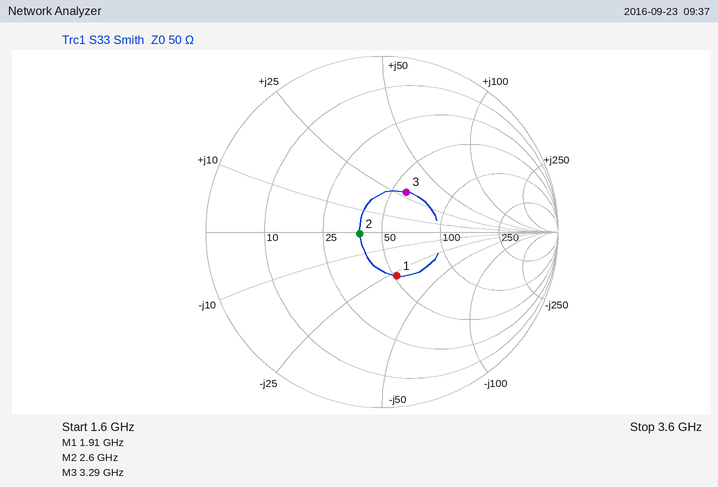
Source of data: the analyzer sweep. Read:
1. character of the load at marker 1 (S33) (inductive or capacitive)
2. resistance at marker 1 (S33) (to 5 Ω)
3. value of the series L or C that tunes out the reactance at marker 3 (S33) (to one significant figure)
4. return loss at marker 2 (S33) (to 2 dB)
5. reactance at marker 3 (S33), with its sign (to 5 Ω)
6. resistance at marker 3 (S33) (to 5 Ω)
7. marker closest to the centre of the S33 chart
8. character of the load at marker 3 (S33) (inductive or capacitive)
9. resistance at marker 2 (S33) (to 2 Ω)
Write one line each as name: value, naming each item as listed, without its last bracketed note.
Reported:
character of the load at marker 1 (S33): capacitive
resistance at marker 1 (S33): 50 Ω
value of the series L or C that tunes out the reactance at marker 3 (S33): 2 pF
return loss at marker 2 (S33): 18 dB
reactance at marker 3 (S33), with its sign: +30 Ω
resistance at marker 3 (S33): 60 Ω
marker closest to the centre of the S33 chart: marker 2
character of the load at marker 3 (S33): inductive
resistance at marker 2 (S33): 38 Ω
